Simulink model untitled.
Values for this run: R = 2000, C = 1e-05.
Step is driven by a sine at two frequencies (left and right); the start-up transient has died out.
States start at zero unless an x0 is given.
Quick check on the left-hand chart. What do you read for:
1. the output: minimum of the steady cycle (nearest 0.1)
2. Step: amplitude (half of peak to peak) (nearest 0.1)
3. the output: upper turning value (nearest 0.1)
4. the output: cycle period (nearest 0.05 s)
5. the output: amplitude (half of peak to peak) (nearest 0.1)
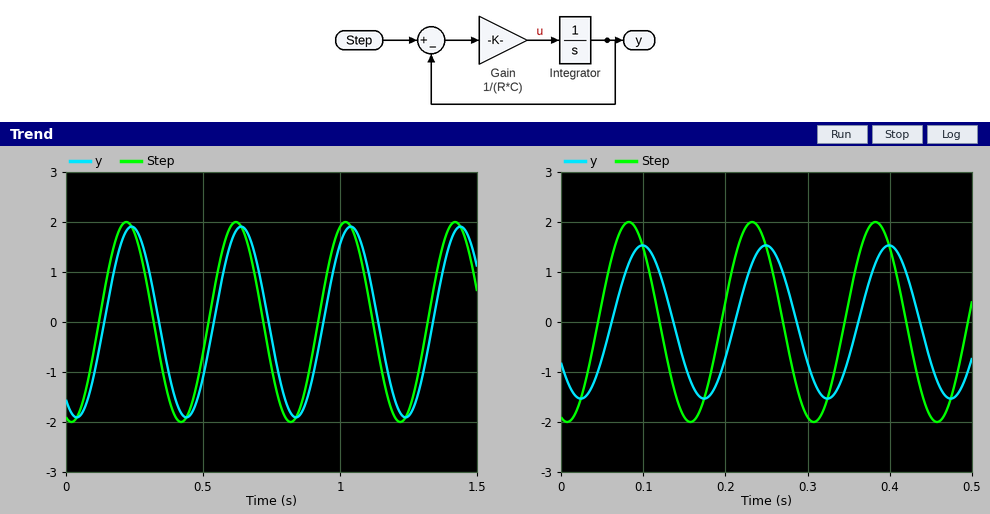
-1.9
2.0
1.9
0.40 s
1.9
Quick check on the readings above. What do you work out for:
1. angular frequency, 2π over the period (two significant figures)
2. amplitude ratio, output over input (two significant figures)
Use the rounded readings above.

16 rad/s
0.95
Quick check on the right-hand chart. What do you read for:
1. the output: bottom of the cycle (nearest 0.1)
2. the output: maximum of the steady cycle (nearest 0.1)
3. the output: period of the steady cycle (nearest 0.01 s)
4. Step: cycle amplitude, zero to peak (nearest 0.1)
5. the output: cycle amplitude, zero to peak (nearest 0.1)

-1.5
1.5
0.15 s
2.0
1.5
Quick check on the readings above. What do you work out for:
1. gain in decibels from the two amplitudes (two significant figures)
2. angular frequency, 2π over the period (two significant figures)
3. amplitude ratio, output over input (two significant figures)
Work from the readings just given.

-2.5 dB
42 rad/s
0.75
